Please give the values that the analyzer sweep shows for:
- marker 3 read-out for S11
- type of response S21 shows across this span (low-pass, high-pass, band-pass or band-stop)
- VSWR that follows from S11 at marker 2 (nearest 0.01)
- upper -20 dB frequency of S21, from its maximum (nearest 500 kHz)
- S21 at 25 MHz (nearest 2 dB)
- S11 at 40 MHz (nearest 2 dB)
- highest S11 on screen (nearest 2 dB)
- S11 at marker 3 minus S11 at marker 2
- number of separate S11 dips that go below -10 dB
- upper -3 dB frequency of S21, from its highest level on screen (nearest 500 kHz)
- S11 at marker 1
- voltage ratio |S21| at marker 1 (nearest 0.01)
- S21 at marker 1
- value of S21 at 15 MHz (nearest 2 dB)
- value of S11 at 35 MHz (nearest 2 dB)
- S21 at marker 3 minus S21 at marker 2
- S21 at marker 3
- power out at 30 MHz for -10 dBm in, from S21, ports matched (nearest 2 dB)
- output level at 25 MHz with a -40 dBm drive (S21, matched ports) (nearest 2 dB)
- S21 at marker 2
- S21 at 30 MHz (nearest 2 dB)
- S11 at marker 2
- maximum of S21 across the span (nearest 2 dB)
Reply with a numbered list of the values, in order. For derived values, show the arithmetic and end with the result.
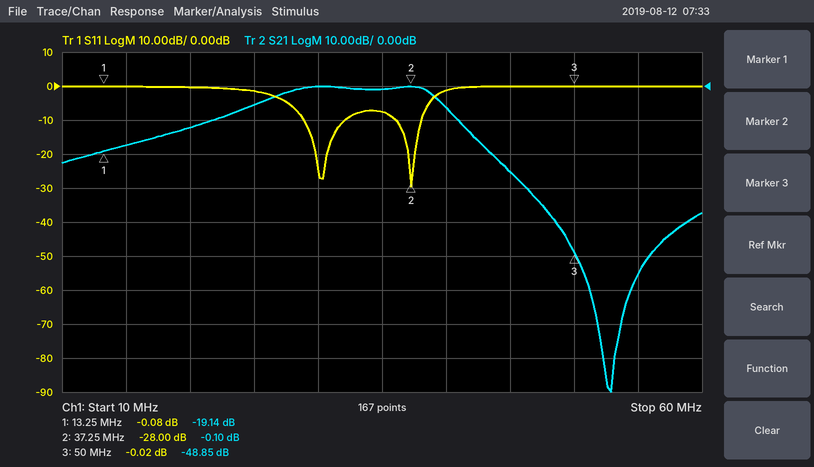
1. -0.02 dB
2. band-pass
3. (1 + 0.0398)/(1 − 0.0398) ≈ 1.08
4. 43.5 MHz
5. -6 dB
6. -2 dB
7. 0 dB
8. -0.02 − (-28) = 27.98 dB
9. 2
10. 39.0 MHz
11. -0.08 dB
12. 10^(-19.14/20) ≈ 0.11
13. -19.14 dB
14. -18 dB
15. -8 dB
16. -48.85 − (-0.1) = -48.75 dB
17. -48.85 dB
18. -10 dBm + (0 dB) = -10 dBm
19. -40 dBm + (-6 dB) = -46 dBm
20. -0.10 dB
21. 0 dB
22. -28.00 dB
23. 0 dB
